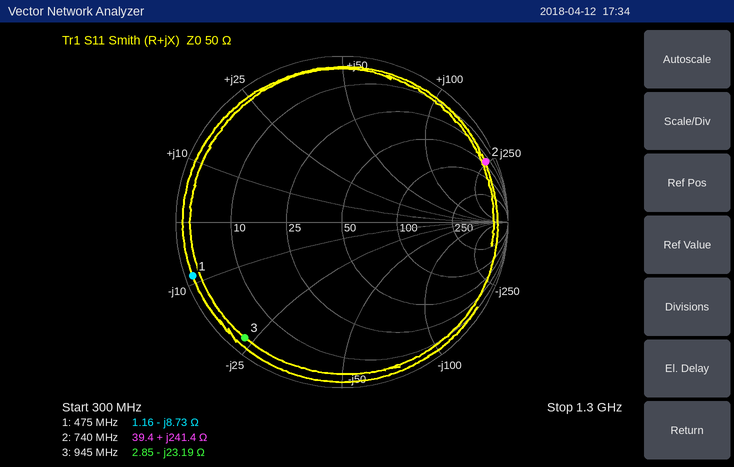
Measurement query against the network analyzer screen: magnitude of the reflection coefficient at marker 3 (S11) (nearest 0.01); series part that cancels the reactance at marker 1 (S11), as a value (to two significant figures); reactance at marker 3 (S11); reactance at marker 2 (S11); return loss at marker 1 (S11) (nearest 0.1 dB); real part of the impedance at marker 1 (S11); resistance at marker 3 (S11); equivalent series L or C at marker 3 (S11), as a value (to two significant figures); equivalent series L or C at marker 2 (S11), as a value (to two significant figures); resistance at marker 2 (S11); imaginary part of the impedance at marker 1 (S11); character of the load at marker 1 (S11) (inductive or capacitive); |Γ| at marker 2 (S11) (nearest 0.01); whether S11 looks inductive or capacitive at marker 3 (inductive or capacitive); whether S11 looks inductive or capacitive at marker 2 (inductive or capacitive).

0.91
2.9 nH
-23.19 Ω
+241.4 Ω
0.4 dB
1.16 Ω
2.85 Ω
7.3 pF
52 nH
39.4 Ω
-8.73 Ω
capacitive
0.94
capacitive
inductive
